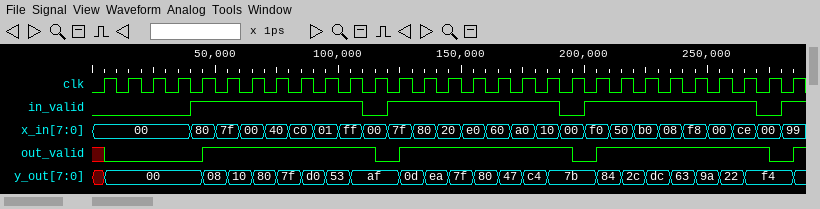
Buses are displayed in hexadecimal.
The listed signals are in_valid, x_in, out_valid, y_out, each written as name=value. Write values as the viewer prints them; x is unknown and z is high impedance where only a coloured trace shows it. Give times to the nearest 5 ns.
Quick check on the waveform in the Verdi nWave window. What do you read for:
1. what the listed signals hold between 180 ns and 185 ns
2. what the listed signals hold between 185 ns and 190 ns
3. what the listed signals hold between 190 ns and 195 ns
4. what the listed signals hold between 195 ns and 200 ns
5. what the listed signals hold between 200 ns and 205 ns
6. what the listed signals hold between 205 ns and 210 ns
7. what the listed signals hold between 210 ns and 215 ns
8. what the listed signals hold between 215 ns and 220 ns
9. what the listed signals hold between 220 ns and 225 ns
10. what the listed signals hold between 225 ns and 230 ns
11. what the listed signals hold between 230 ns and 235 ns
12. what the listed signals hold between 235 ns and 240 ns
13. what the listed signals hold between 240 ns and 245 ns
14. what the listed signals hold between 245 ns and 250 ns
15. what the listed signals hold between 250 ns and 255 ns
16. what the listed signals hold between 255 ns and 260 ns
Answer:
in_valid=1, x_in=10, out_valid=1, y_out=c4
in_valid=1, x_in=10, out_valid=1, y_out=7b
in_valid=0, x_in=00, out_valid=1, y_out=7b
in_valid=0, x_in=00, out_valid=0, y_out=7b
in_valid=1, x_in=f0, out_valid=0, y_out=7b
in_valid=1, x_in=f0, out_valid=1, y_out=84
in_valid=1, x_in=50, out_valid=1, y_out=84
in_valid=1, x_in=50, out_valid=1, y_out=2c
in_valid=1, x_in=b0, out_valid=1, y_out=2c
in_valid=1, x_in=b0, out_valid=1, y_out=dc
in_valid=1, x_in=08, out_valid=1, y_out=dc
in_valid=1, x_in=08, out_valid=1, y_out=63
in_valid=1, x_in=f8, out_valid=1, y_out=63
in_valid=1, x_in=f8, out_valid=1, y_out=9a
in_valid=1, x_in=00, out_valid=1, y_out=9a
in_valid=1, x_in=00, out_valid=1, y_out=22
